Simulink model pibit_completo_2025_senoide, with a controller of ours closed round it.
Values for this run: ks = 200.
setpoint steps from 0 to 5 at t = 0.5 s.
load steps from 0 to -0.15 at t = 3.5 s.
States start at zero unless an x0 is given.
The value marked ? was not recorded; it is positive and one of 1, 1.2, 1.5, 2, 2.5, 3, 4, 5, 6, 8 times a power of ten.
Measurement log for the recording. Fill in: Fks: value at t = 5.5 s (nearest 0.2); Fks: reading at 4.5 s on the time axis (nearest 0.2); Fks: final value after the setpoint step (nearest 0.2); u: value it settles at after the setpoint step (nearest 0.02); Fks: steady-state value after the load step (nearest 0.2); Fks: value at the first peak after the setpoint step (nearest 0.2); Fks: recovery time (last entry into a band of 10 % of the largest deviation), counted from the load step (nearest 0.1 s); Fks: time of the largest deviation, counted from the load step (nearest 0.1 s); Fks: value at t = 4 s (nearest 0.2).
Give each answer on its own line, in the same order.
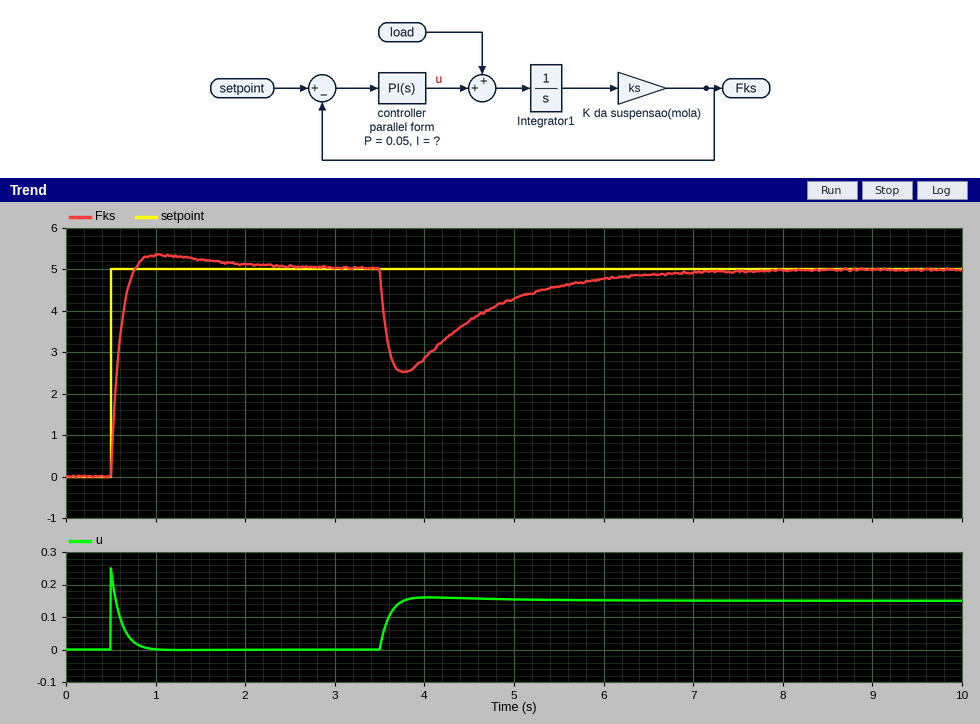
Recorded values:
4.6
3.8
5.0
0.00
5.0
5.4
2.4 s
0.3 s
2.8
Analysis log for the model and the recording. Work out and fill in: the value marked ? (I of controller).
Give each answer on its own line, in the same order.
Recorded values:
0.05
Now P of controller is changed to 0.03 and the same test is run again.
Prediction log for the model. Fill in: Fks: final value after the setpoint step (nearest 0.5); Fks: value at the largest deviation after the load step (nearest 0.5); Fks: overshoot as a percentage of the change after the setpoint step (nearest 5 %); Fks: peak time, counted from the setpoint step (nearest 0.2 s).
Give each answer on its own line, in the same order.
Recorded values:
5.0
1.5
15 %
0.6 s
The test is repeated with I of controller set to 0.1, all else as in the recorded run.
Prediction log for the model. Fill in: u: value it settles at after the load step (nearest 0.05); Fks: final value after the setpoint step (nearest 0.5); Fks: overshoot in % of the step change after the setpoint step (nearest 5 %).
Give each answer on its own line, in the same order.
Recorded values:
0.15
5.0
10 %
